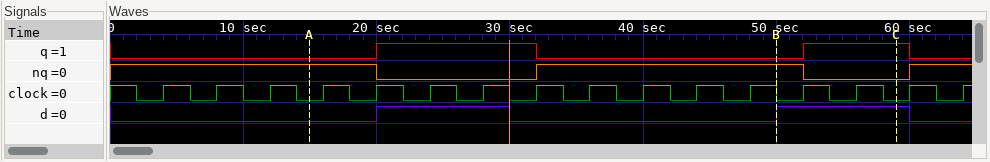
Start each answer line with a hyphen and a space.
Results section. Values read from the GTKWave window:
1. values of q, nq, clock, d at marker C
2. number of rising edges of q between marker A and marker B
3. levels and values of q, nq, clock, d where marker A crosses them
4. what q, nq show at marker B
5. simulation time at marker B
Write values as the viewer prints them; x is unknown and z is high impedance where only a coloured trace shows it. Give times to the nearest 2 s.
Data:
- q=1, nq=0, clock=0, d=1
- 1
- q=0, nq=1, clock=0, d=0
- q=0, nq=1
- 50 s
